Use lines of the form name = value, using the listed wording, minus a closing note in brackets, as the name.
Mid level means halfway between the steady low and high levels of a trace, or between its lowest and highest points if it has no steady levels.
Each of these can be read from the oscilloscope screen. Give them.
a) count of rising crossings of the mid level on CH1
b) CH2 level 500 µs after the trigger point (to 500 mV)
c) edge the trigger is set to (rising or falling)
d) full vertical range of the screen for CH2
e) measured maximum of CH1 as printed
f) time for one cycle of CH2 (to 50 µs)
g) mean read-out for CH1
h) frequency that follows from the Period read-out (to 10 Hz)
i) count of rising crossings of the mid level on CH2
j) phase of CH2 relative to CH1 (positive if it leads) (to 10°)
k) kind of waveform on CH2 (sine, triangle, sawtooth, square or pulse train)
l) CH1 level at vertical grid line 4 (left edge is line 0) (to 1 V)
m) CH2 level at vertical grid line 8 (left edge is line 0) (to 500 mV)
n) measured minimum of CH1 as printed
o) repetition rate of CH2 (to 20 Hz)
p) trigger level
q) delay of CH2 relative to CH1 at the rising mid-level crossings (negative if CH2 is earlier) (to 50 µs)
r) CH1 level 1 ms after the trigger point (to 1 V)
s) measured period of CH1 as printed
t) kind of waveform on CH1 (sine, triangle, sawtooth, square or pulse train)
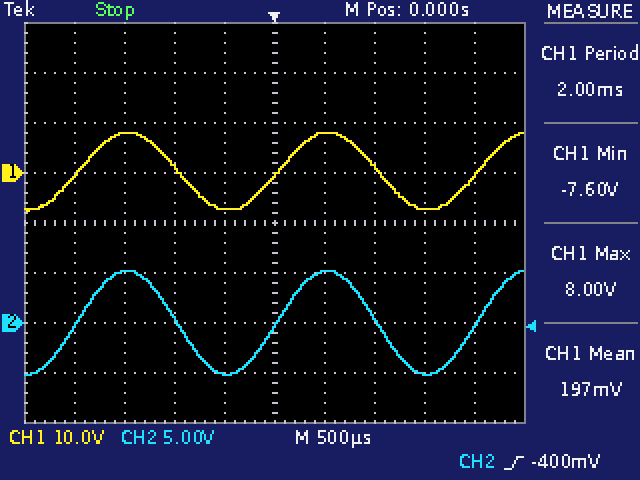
count of rising crossings of the mid level on CH1 = 3
CH2 level 500 µs after the trigger point = 5.0 V
edge the trigger is set to = rising
full vertical range of the screen for CH2 = 40 V
measured maximum of CH1 as printed = 8.00 V
time for one cycle of CH2 = 2.00 ms
mean read-out for CH1 = 197 mV
frequency that follows from the Period read-out = 500 Hz
count of rising crossings of the mid level on CH2 = 3
phase of CH2 relative to CH1 (positive if it leads) = 0°
kind of waveform on CH2 = sine
CH1 level at vertical grid line 4 (left edge is line 0) = -7 V
CH2 level at vertical grid line 8 (left edge is line 0) = -5.0 V
measured minimum of CH1 as printed = -7.60 V
repetition rate of CH2 = 500 Hz
trigger level = -400 mV
delay of CH2 relative to CH1 at the rising mid-level crossings (negative if CH2 is earlier) = 0 µs
CH1 level 1 ms after the trigger point = 1 V
measured period of CH1 as printed = 2.00 ms
kind of waveform on CH1 = sine
